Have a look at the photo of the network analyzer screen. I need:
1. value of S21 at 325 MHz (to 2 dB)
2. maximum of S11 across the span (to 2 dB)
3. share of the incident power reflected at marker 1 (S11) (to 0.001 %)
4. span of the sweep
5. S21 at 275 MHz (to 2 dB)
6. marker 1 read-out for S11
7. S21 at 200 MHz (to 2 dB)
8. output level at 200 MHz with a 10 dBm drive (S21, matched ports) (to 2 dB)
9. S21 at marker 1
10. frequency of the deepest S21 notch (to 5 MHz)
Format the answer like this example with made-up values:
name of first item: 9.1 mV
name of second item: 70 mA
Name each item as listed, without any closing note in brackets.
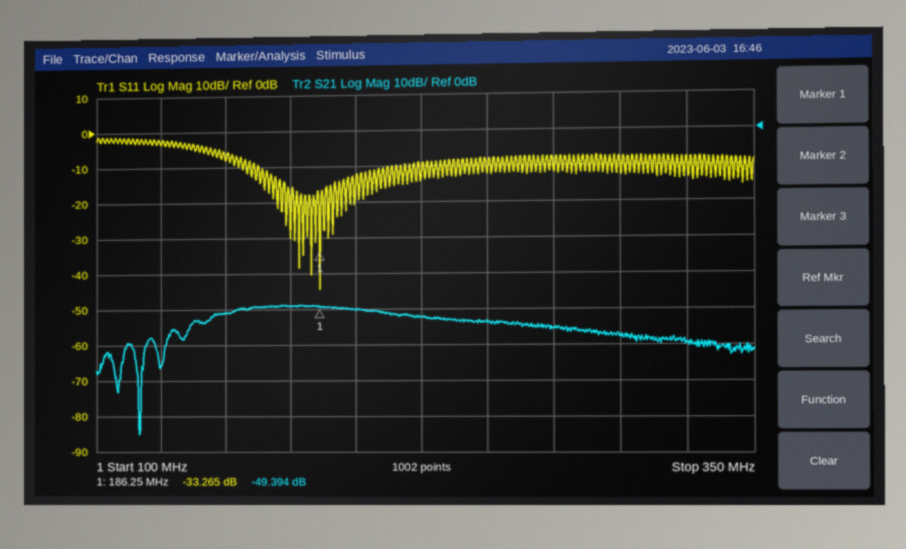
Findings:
value of S21 at 325 MHz: -60 dB
maximum of S11 across the span: -2 dB
share of the incident power reflected at marker 1 (S11): 0.047 %
span of the sweep: 250 MHz
S21 at 275 MHz: -56 dB
marker 1 read-out for S11: -33.265 dB
S21 at 200 MHz: -50 dB
output level at 200 MHz with a 10 dBm drive (S21, matched ports): -40 dBm
S21 at marker 1: -49.394 dB
frequency of the deepest S21 notch: 115 MHz
